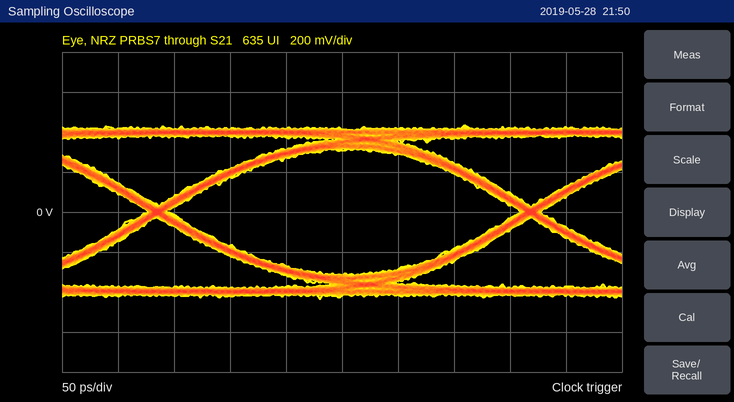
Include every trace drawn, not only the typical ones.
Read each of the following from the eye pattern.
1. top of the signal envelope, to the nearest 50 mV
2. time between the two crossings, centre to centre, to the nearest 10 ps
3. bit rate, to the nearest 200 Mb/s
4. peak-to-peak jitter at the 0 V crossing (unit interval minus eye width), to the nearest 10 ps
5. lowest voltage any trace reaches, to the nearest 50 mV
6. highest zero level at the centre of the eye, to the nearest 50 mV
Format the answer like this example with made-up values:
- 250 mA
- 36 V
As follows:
- 450 mV
- 330 ps
- 3.0 Gb/s
- 20 ps
- -450 mV
- -300 mV
